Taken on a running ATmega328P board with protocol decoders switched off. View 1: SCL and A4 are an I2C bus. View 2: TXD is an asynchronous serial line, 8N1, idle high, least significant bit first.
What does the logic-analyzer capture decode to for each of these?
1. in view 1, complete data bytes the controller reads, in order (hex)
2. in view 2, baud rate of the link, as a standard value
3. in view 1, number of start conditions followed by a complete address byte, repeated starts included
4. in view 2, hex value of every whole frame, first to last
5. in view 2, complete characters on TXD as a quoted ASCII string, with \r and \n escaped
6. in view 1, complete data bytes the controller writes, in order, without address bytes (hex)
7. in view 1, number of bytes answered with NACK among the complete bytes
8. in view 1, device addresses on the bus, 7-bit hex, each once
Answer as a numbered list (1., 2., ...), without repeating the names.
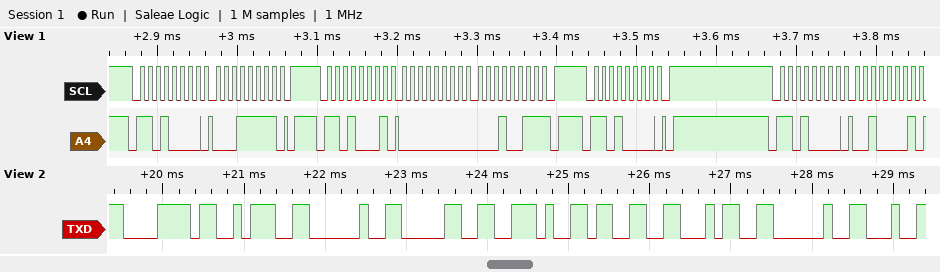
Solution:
1. 00 13
2. 9600 baud
3. 4
4. 0x78 0x3A 0x20 0x30 0x2E 0x33 0x34 0x20
5. "x: 0.34 "
6. 1F 21
7. 1
8. 0x68
